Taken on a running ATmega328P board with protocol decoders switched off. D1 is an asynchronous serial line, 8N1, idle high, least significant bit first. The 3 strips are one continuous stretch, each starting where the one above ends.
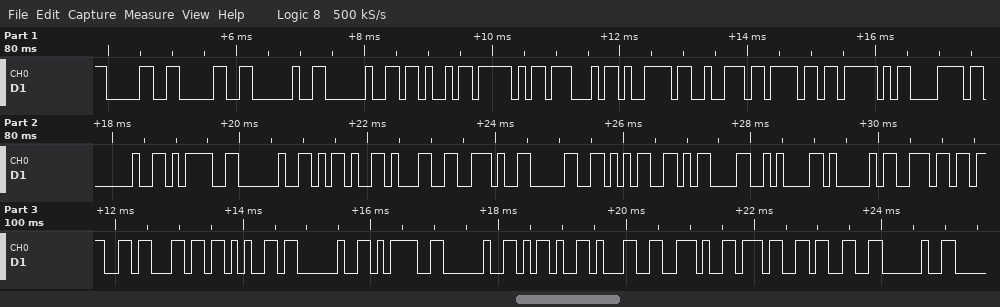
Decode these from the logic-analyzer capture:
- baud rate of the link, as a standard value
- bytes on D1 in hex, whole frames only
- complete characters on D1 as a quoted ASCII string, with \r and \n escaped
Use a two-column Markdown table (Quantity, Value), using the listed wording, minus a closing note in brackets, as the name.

| Quantity | Value |
|---|---|
| baud rate of the link, as a standard value | 9600 baud |
| bytes on D1 in hex, whole frames only | 30 30 20 20 4B 5F 47 79 72 6F 5F 78 20 3D 20 2D 31 2E 30 35 0D 0A 41 6E 67 6C 65 20 3D 20 2D 31 2E 37 33 20 |
| complete characters on D1 as a quoted ASCII string, with \r and \n escaped | "00  K_Gyro_x = -1.05\r\nAngle = -1.73 " |
